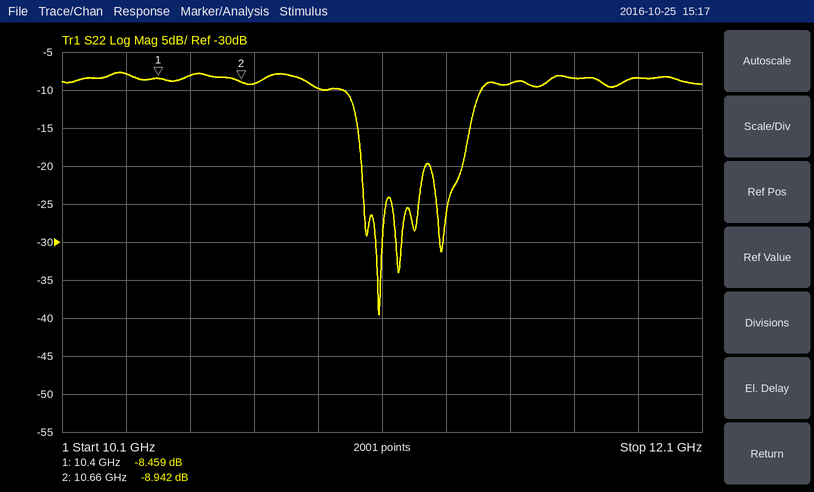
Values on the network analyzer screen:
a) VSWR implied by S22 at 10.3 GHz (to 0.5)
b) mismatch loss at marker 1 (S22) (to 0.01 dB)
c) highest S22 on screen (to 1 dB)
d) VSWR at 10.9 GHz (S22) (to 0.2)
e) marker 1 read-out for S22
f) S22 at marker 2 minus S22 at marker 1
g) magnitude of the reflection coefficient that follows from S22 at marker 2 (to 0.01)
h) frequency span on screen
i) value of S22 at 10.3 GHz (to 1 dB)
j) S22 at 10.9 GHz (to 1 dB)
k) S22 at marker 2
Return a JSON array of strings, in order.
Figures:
["2.5", "0.67 dB", "-8 dB", "2.0", "-8.459 dB", "-0.483 dB", "0.36", "2 GHz", "-8 dB", "-10 dB", "-8.942 dB"]
